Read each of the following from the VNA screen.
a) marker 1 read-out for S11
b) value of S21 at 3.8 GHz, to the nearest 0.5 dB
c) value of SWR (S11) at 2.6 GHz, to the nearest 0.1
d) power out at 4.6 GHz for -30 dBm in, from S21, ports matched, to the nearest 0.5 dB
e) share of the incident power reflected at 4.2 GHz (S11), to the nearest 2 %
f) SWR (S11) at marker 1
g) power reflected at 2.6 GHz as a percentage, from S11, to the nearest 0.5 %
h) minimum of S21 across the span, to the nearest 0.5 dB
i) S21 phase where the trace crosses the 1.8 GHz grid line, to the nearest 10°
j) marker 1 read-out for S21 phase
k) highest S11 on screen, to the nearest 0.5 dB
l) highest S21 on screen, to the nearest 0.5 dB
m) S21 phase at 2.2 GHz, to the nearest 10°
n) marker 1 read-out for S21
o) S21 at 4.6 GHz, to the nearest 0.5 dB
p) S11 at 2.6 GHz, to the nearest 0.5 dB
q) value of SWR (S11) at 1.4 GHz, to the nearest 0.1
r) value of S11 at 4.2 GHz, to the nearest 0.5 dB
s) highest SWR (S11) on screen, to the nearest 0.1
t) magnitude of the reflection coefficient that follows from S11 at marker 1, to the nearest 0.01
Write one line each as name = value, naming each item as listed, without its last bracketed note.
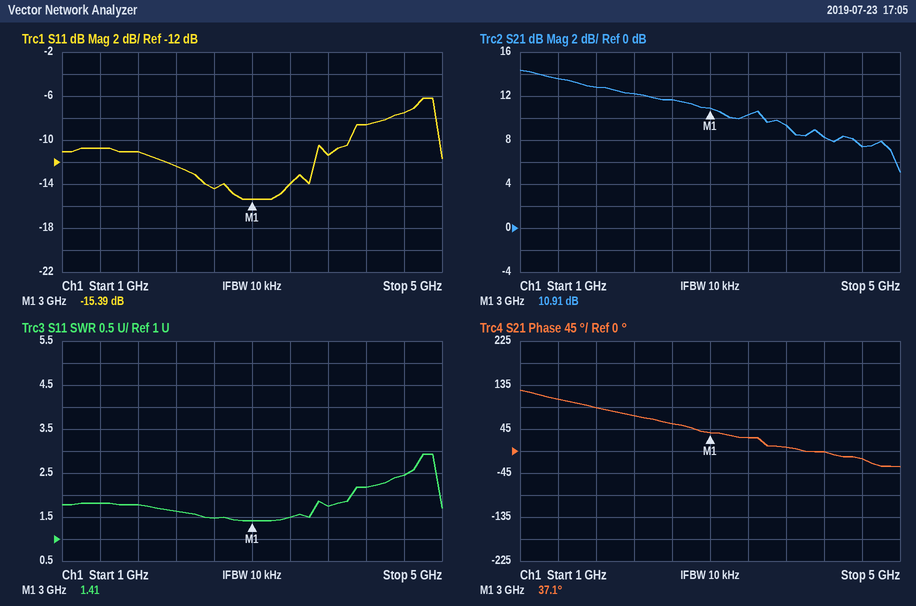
marker 1 read-out for S11 = -15.39 dB
value of S21 at 3.8 GHz, to the nearest 0.5 dB = 9.5 dB
value of SWR (S11) at 2.6 GHz, to the nearest 0.1 = 1.5
power out at 4.6 GHz for -30 dBm in, from S21, ports matched, to the nearest 0.5 dB = -22.5 dBm
share of the incident power reflected at 4.2 GHz (S11), to the nearest 2 % = 14 %
SWR (S11) at marker 1 = 1.41
power reflected at 2.6 GHz as a percentage, from S11, to the nearest 0.5 % = 3.5 %
minimum of S21 across the span, to the nearest 0.5 dB = 5.0 dB
S21 phase where the trace crosses the 1.8 GHz grid line, to the nearest 10° = 90°
marker 1 read-out for S21 phase = 37.1°
highest S11 on screen, to the nearest 0.5 dB = -6.0 dB
highest S21 on screen, to the nearest 0.5 dB = 14.5 dB
S21 phase at 2.2 GHz, to the nearest 10° = 70°
marker 1 read-out for S21 = 10.91 dB
S21 at 4.6 GHz, to the nearest 0.5 dB = 7.5 dB
S11 at 2.6 GHz, to the nearest 0.5 dB = -14.5 dB
value of SWR (S11) at 1.4 GHz, to the nearest 0.1 = 1.8
value of S11 at 4.2 GHz, to the nearest 0.5 dB = -8.5 dB
highest SWR (S11) on screen, to the nearest 0.1 = 2.9
magnitude of the reflection coefficient that follows from S11 at marker 1, to the nearest 0.01 = 0.17
